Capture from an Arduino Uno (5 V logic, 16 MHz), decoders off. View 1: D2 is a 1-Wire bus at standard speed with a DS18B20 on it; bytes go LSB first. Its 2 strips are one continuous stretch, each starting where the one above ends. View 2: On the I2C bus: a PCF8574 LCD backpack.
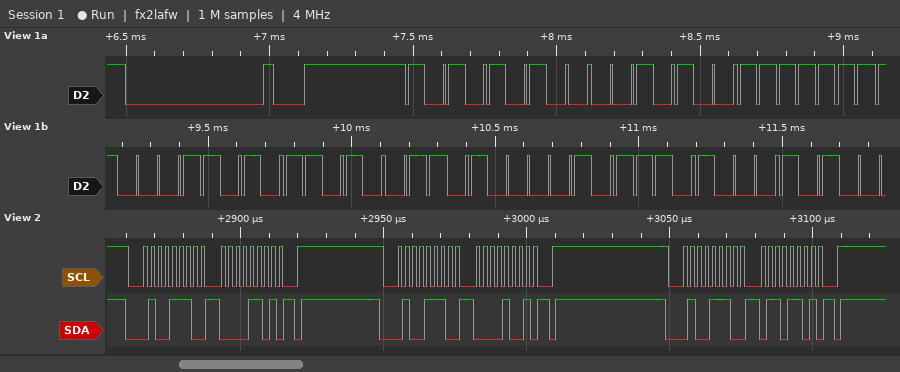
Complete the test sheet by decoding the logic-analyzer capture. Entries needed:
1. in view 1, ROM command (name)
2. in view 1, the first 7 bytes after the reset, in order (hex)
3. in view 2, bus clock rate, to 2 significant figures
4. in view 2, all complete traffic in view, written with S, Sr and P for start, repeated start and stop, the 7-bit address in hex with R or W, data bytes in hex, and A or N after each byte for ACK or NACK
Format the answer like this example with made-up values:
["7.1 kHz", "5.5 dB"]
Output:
["Match ROM", "55 28 FF 58 CB 42 17", "400 kHz", "S 27W A 0D A P S 27W A 09 A P S 27W A 6D A P"]
